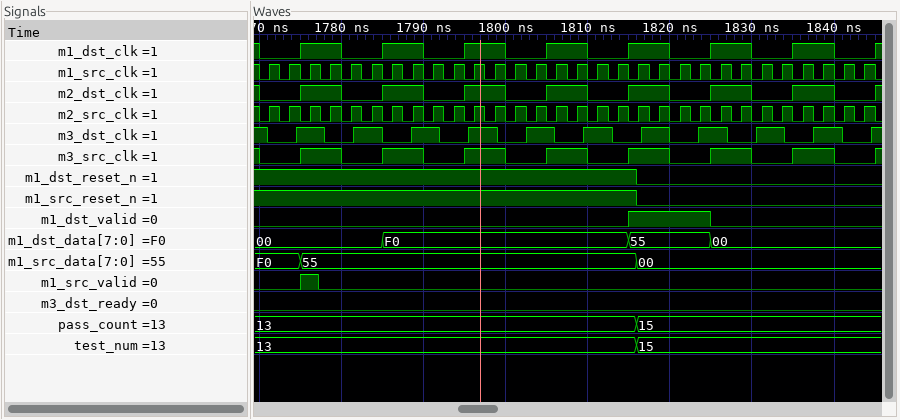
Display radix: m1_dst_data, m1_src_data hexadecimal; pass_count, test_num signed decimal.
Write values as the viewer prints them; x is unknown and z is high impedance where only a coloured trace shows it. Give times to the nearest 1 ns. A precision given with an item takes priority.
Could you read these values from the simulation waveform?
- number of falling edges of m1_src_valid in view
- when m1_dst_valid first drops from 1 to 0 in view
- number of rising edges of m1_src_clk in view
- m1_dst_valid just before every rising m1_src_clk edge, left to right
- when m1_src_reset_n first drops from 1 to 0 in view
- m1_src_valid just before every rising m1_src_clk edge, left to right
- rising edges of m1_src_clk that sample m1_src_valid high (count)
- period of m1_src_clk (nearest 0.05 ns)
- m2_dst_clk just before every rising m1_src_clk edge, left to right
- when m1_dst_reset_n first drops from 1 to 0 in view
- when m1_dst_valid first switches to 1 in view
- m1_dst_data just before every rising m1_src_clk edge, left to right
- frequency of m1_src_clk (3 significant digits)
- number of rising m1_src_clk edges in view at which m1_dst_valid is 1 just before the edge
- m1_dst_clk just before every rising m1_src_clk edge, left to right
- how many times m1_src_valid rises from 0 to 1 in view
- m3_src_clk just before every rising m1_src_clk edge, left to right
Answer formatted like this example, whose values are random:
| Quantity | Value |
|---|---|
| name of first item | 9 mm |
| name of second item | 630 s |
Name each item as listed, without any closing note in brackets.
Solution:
| Quantity | Value |
|---|---|
| number of falling edges of m1_src_valid in view | 1 |
| when m1_dst_valid first drops from 1 to 0 in view | 1825 ns |
| number of rising edges of m1_src_clk in view | 30 |
| m1_dst_valid just before every rising m1_src_clk edge, left to right | 0 0 0 0 0 0 0 0 0 0 0 0 0 0 0 0 0 0 1 1 1 1 0 0 0 0 0 0 0 0 |
| when m1_src_reset_n first drops from 1 to 0 in view | 1816 ns |
| m1_src_valid just before every rising m1_src_clk edge, left to right | 0 0 1 0 0 0 0 0 0 0 0 0 0 0 0 0 0 0 0 0 0 0 0 0 0 0 0 0 0 0 |
| rising edges of m1_src_clk that sample m1_src_valid high | 1 |
| period of m1_src_clk | 2.5 ns |
| m2_dst_clk just before every rising m1_src_clk edge, left to right | 0 0 1 1 0 0 1 1 0 0 1 1 0 0 1 1 0 0 1 1 0 0 1 1 0 0 1 1 0 0 |
| when m1_dst_reset_n first drops from 1 to 0 in view | 1816 ns |
| when m1_dst_valid first switches to 1 in view | 1815 ns |
| m1_dst_data just before every rising m1_src_clk edge, left to right | 00, 00, 00, 00, 00, 00, F0, F0, F0, F0, F0, F0, F0, F0, F0, F0, F0, F0, 55, 55, 55, 55, 00, 00, 00, 00, 00, 00, 00, 00 |
| frequency of m1_src_clk | 400 MHz |
| number of rising m1_src_clk edges in view at which m1_dst_valid is 1 just before the edge | 4 |
| m1_dst_clk just before every rising m1_src_clk edge, left to right | 0 0 1 1 0 0 1 1 0 0 1 1 0 0 1 1 0 0 1 1 0 0 1 1 0 0 1 1 0 0 |
| how many times m1_src_valid rises from 0 to 1 in view | 1 |
| m3_src_clk just before every rising m1_src_clk edge, left to right | 0 0 1 1 0 0 1 1 0 0 1 1 0 0 1 1 0 0 1 1 0 0 1 1 0 0 1 1 0 0 |
